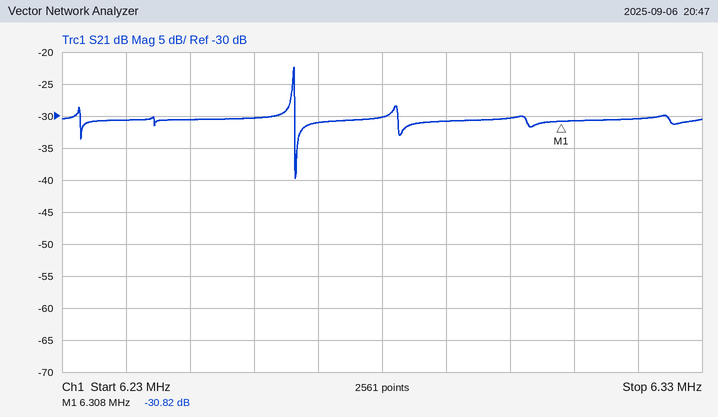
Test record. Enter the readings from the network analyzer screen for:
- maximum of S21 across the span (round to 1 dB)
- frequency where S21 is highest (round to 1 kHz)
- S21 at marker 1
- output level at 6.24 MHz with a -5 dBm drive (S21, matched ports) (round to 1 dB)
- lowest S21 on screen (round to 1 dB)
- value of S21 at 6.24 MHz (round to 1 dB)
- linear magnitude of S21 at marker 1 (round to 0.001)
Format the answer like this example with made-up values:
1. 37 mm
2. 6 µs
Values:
1. -22 dB
2. 6.266 MHz
3. -30.82 dB
4. -36 dBm
5. -40 dB
6. -31 dB
7. 0.029
